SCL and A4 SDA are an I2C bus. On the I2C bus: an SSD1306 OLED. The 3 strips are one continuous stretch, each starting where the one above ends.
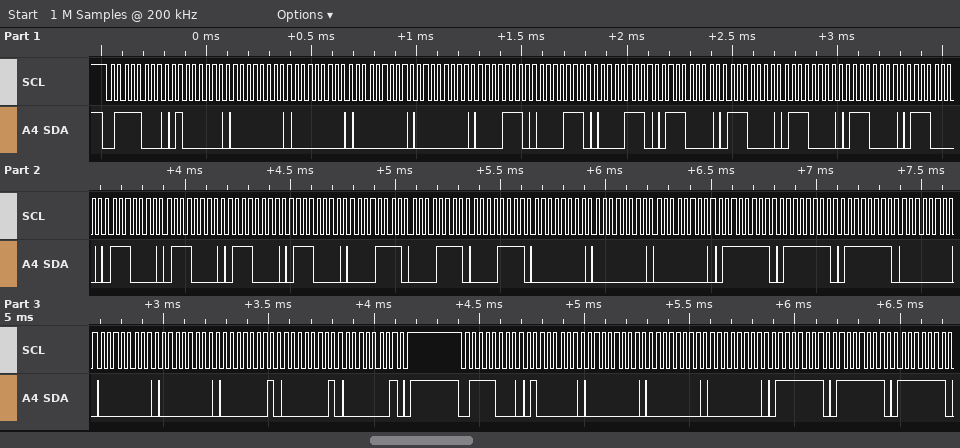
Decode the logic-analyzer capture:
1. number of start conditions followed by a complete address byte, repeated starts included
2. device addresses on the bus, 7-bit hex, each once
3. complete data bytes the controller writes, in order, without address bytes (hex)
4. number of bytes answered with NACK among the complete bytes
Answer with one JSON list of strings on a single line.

["2", "0x3C", "40 00 00 00 00 0E 0E 0E 70 70 70 70 70 70 70 70 70 0F 0F 0F 00 00 00 7F 7F 7F 00 00 00 01 01 01 40 00 00 00 7F 7F 7F", "0"]
